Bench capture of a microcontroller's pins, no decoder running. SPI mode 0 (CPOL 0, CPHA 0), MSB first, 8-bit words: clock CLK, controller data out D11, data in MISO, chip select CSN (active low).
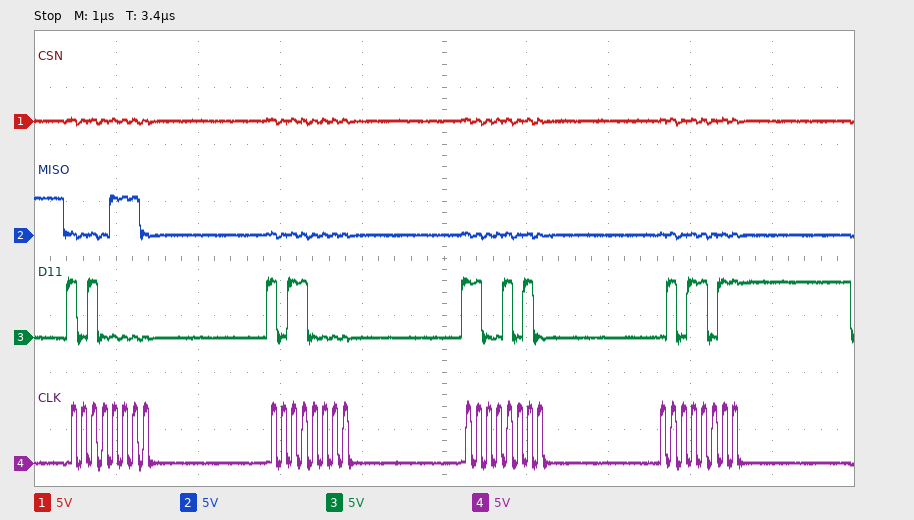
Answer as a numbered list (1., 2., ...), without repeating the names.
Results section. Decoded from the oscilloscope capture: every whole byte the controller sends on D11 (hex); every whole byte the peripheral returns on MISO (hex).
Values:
1. 0xA0 0xB0 0xCA 0x5B
2. 0x0E 0x00 0x00 0x00
